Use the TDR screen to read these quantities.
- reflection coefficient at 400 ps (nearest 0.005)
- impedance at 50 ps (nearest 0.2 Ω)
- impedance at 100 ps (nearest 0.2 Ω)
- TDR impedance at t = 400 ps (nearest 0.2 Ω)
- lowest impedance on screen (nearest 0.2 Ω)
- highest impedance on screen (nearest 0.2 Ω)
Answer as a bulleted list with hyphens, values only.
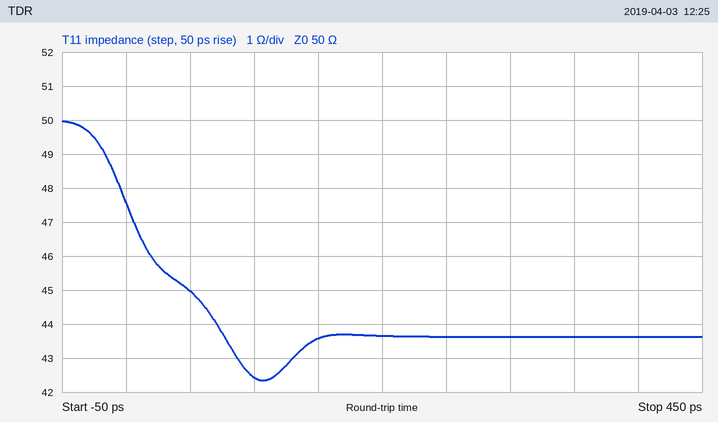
- -0.070
- 45.0 Ω
- 42.4 Ω
- 43.6 Ω
- 42.4 Ω
- 50.0 Ω
